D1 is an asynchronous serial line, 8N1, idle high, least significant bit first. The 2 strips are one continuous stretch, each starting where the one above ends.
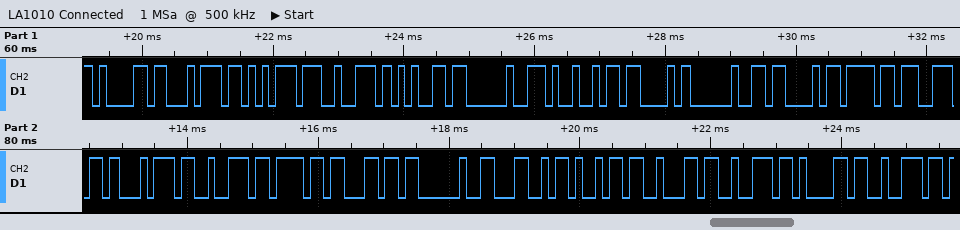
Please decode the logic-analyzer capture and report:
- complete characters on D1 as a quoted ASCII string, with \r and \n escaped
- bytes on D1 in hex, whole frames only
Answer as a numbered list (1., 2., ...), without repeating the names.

1. "ature IC Control Librar"
2. 61 74 75 72 65 20 49 43 20 43 6F 6E 74 72 6F 6C 20 4C 69 62 72 61 72
